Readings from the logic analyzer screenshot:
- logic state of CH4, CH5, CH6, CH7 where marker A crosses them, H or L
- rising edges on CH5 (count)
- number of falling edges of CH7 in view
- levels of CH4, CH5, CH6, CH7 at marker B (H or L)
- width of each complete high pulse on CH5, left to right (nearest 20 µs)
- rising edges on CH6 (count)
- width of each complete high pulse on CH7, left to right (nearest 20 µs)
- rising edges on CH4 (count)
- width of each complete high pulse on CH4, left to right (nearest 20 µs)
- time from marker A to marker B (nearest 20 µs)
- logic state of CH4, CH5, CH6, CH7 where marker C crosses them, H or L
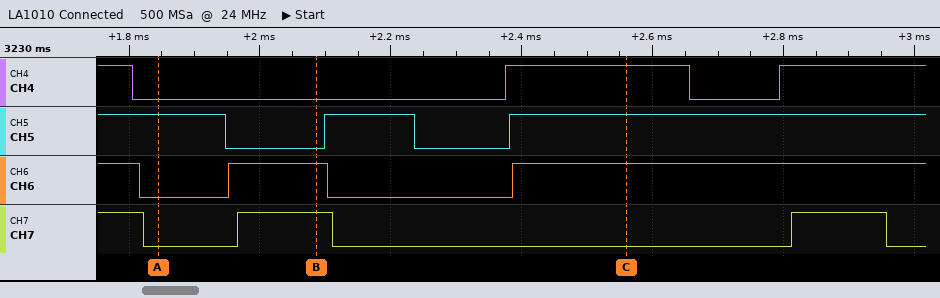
CH4=L, CH5=H, CH6=L, CH7=L
2
3
CH4=L, CH5=L, CH6=H, CH7=H
140 µs
2
140 µs, 140 µs
2
280 µs
240 µs
CH4=H, CH5=H, CH6=H, CH7=L
